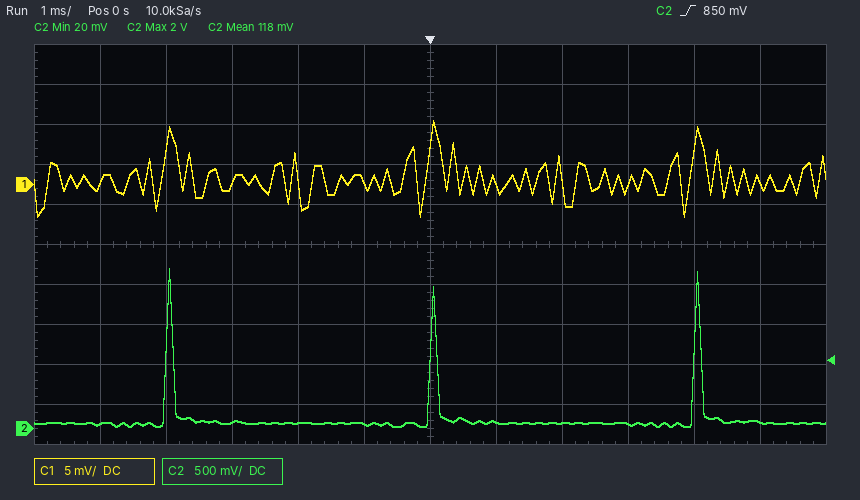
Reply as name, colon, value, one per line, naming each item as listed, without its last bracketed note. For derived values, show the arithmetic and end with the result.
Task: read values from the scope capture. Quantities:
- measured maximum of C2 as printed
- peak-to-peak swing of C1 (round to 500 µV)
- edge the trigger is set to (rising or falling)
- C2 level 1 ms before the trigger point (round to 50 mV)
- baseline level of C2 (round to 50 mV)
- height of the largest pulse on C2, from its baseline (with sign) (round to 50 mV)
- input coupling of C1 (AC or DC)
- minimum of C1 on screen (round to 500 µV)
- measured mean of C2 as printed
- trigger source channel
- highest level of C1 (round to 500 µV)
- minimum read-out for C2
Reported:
measured maximum of C2 as printed: 2 V
peak-to-peak swing of C1: 8.0 mV − (-4.0 mV) = 12.0 mV
edge the trigger is set to: rising
C2 level 1 ms before the trigger point: 50 mV
baseline level of C2: 50 mV
height of the largest pulse on C2, from its baseline (with sign): +1.95 V
input coupling of C1: DC
minimum of C1 on screen: -4.0 mV
measured mean of C2 as printed: 118 mV
trigger source channel: C2
highest level of C1: 8.0 mV
minimum read-out for C2: 20 mV
